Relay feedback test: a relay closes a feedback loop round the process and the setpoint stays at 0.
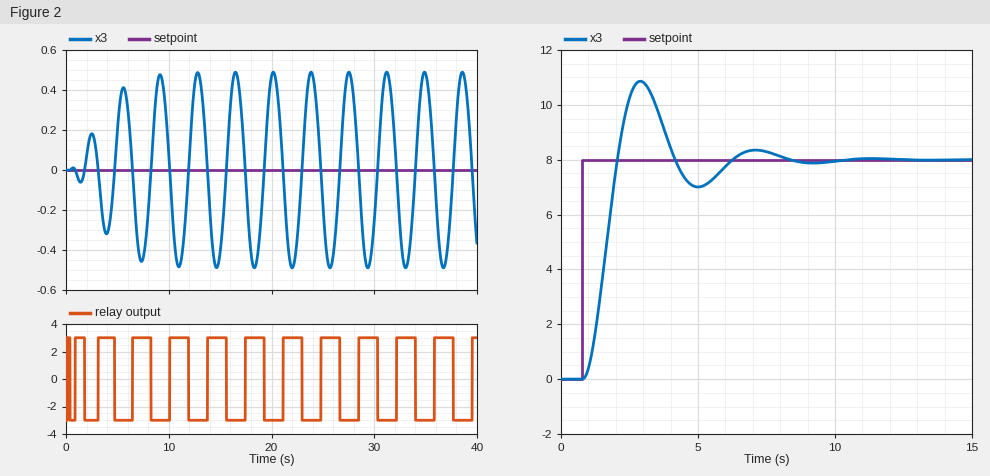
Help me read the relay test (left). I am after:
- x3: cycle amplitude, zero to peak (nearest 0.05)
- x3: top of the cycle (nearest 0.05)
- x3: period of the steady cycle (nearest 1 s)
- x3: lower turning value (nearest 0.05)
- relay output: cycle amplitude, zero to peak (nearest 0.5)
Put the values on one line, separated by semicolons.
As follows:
0.50; 0.50; 4 s; -0.50; 3.0
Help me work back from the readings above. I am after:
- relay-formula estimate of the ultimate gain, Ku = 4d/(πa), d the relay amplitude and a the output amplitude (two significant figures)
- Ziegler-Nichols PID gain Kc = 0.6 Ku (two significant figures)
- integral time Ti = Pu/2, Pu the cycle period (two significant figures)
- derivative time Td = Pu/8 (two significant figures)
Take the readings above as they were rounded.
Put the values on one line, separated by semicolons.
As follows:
7.6; 4.6; 2.0 s; 0.50 s
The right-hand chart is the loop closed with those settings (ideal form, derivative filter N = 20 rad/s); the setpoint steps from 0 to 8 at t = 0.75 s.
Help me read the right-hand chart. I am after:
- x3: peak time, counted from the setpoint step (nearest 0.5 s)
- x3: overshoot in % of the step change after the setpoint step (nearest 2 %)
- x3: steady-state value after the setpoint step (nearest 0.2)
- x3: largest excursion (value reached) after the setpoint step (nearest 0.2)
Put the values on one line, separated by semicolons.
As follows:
2.0 s; 36 %; 8.0; 10.8
